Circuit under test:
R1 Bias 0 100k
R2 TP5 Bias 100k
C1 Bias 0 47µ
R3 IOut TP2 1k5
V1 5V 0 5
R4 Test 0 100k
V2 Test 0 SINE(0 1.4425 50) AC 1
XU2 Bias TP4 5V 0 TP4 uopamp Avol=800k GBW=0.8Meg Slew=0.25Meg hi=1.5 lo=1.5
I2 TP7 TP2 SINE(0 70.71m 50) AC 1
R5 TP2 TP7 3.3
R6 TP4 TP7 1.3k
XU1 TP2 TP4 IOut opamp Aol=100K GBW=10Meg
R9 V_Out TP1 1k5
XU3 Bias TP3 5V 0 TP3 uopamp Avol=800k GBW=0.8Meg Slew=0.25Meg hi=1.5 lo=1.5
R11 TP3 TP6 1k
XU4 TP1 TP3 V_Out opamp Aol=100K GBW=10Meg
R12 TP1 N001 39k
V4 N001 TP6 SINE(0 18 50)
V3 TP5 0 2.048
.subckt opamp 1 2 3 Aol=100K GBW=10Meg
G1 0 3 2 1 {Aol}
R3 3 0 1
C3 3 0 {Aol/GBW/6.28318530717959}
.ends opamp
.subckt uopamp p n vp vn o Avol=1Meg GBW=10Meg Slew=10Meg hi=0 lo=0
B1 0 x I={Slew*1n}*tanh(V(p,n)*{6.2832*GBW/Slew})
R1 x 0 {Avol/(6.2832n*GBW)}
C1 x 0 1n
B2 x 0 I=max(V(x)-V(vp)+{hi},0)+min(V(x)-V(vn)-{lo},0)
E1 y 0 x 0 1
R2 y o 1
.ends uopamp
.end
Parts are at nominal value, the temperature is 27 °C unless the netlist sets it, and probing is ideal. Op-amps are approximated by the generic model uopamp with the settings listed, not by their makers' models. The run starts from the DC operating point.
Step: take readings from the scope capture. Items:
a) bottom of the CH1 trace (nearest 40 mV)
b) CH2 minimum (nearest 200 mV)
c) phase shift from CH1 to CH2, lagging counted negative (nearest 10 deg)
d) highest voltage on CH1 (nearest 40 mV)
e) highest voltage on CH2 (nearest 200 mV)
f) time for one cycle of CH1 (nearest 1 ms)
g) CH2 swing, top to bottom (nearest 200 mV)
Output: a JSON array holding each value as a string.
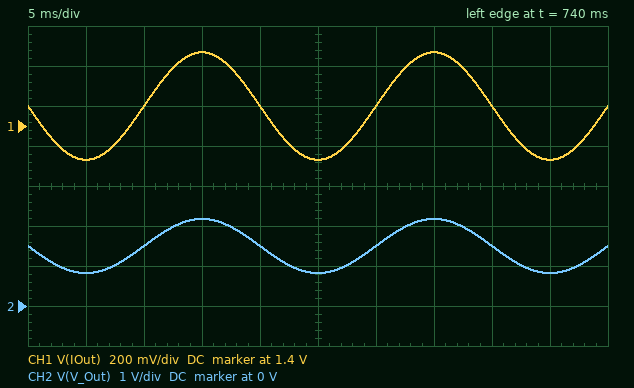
["1.24 V", "800 mV", "0 deg", "1.76 V", "2.2 V", "20 ms", "1.4 V"]
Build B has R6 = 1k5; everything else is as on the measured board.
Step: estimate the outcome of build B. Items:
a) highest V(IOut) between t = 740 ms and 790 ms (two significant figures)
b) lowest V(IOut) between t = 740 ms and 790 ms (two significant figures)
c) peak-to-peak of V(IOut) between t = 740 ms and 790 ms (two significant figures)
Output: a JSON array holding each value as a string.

["1.7 V", "1.3 V", "470 mV"]
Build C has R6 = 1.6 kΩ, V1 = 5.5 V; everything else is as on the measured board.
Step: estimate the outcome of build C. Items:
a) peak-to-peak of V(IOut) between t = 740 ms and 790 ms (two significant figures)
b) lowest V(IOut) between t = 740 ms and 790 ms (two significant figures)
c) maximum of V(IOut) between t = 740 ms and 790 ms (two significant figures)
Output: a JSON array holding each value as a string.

["440 mV", "1.3 V", "1.7 V"]
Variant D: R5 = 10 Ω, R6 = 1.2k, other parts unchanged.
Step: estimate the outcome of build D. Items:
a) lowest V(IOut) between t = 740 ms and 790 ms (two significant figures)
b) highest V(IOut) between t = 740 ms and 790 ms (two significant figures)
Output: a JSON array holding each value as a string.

["620 mV", "2.4 V"]
